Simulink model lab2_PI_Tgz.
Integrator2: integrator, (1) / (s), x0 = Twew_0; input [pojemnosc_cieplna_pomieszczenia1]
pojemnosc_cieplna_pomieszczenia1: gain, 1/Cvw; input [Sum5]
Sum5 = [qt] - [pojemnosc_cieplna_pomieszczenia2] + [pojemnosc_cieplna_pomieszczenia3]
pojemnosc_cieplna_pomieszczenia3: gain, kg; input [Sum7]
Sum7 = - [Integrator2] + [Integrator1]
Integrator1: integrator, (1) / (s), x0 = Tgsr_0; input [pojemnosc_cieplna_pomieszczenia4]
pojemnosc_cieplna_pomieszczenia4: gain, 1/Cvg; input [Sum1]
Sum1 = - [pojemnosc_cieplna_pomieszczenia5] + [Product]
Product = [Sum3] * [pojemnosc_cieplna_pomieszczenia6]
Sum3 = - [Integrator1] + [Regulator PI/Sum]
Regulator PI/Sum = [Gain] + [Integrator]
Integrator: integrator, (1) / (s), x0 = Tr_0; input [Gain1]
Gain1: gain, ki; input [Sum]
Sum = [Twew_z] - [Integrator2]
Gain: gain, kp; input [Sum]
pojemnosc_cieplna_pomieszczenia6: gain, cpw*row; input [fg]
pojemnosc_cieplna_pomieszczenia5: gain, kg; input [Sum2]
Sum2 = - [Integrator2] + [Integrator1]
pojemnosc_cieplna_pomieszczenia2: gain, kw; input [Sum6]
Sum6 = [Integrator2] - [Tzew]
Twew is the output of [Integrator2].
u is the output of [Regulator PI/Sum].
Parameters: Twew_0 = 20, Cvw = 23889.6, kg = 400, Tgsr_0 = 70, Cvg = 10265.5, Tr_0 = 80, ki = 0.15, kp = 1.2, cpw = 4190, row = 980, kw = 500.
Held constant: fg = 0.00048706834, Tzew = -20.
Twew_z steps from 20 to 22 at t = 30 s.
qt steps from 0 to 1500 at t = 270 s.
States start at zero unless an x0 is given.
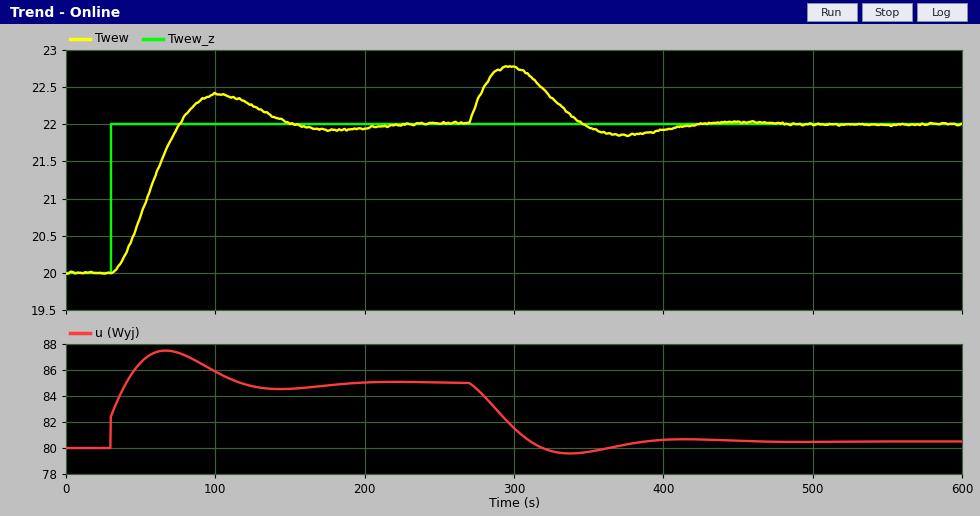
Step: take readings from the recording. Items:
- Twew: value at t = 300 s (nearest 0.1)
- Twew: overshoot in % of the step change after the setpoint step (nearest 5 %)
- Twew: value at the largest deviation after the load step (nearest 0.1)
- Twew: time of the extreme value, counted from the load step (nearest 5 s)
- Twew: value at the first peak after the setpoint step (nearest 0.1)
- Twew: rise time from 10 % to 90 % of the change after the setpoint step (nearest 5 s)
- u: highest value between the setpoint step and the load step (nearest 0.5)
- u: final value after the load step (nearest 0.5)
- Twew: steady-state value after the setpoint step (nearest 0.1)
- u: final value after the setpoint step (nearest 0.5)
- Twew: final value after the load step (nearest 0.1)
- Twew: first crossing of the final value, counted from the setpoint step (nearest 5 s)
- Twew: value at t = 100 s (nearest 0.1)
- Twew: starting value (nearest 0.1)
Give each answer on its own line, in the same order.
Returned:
22.8
20 %
22.8
25 s
22.4
30 s
87.5
80.5
22.0
85.0
22.0
45 s
22.4
20.0
